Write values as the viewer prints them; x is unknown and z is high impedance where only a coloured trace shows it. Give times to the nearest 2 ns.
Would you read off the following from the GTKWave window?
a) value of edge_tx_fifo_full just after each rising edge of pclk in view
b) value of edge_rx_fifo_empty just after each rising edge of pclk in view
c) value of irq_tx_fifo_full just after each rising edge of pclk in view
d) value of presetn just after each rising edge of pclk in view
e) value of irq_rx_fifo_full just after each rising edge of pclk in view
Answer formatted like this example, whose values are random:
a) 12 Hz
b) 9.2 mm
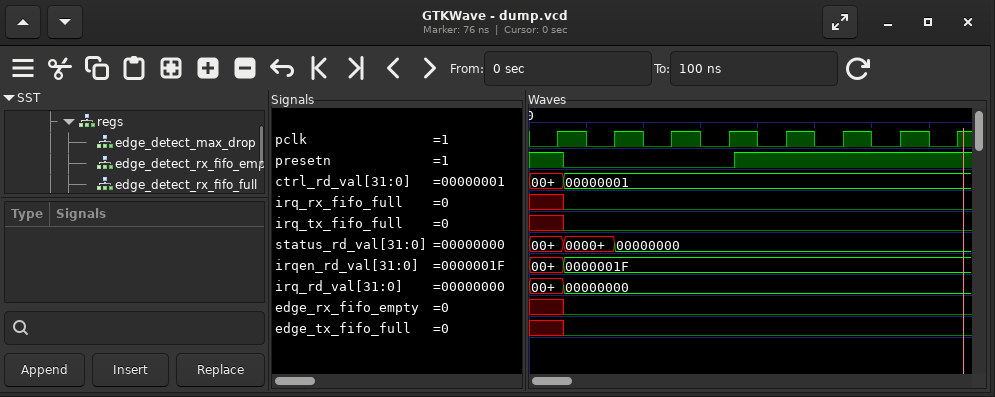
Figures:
a) x 0 0 0 0 0 0 0
b) x 0 0 0 0 0 0 0
c) x 0 0 0 0 0 0 0
d) 1 0 0 0 1 1 1 1
e) x 0 0 0 0 0 0 0
